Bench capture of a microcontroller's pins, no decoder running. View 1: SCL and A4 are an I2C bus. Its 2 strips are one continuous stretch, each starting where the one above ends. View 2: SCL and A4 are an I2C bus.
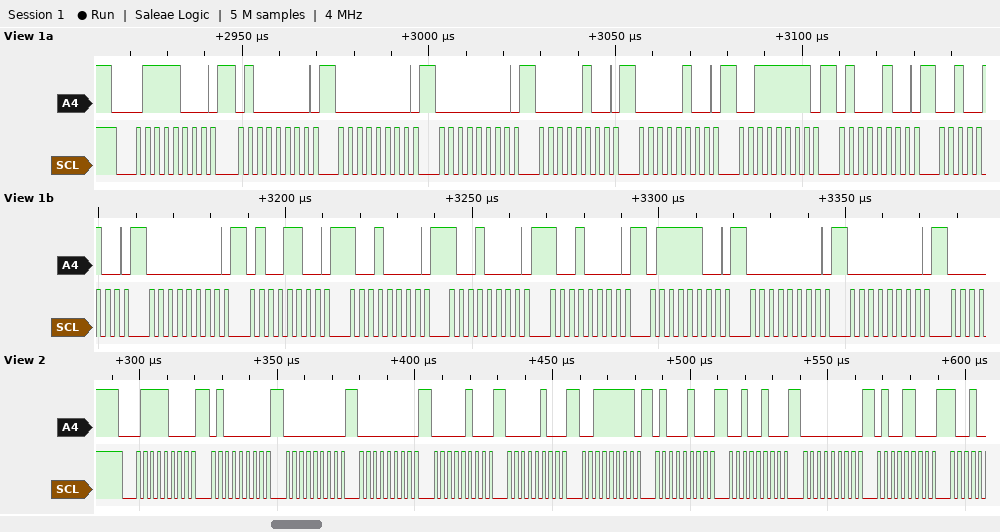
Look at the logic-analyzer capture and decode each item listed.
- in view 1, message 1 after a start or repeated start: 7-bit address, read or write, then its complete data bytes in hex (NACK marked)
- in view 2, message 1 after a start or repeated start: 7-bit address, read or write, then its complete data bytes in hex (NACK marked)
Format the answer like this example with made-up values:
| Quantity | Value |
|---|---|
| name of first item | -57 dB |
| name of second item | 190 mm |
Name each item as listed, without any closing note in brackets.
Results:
| Quantity | Value |
|---|---|
| in view 1, message 1 after a start or repeated start: 7-bit address, read or write, then its complete data bytes in hex | 0x3C write: 40 00 00 04 04 3F 44 24 00 4C 90 90 90 7C 00 00 |
| in view 2, message 1 after a start or repeated start: 7-bit address, read or write, then its complete data bytes in hex | 0x3C write: 40 00 00 04 04 3F 44 24 00 4C |
